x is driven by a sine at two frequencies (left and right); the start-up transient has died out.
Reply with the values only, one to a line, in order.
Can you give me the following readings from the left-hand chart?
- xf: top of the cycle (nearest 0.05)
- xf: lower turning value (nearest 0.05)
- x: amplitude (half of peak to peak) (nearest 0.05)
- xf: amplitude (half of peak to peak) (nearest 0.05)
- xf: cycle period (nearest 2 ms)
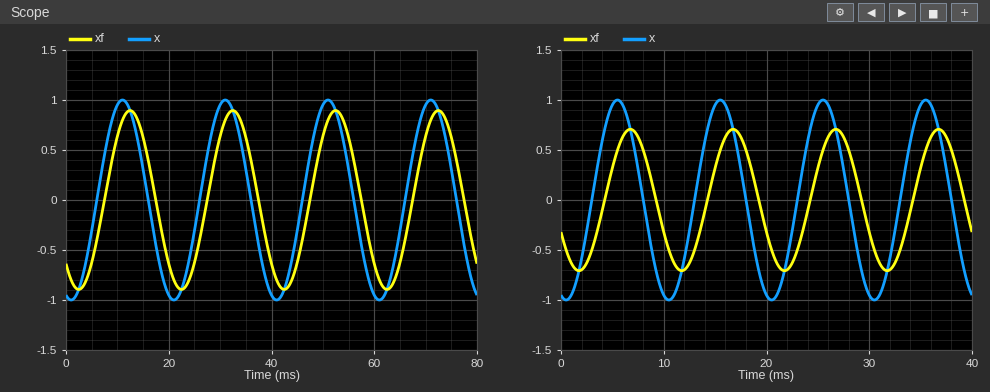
0.90
-0.90
1.00
0.90
20 ms
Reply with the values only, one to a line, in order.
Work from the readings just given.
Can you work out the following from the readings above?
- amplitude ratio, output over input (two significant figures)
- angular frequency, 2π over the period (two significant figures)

0.90
0.31 rad/ms
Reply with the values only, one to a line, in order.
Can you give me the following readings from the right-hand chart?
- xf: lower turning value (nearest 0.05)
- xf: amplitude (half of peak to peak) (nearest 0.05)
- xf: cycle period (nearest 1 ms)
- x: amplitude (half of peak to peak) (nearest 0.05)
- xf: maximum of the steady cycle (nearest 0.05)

-0.70
0.70
10 ms
1.00
0.70
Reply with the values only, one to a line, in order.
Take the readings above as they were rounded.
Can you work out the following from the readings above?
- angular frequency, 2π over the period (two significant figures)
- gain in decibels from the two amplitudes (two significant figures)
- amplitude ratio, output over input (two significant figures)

0.63 rad/ms
-3.1 dB
0.70
